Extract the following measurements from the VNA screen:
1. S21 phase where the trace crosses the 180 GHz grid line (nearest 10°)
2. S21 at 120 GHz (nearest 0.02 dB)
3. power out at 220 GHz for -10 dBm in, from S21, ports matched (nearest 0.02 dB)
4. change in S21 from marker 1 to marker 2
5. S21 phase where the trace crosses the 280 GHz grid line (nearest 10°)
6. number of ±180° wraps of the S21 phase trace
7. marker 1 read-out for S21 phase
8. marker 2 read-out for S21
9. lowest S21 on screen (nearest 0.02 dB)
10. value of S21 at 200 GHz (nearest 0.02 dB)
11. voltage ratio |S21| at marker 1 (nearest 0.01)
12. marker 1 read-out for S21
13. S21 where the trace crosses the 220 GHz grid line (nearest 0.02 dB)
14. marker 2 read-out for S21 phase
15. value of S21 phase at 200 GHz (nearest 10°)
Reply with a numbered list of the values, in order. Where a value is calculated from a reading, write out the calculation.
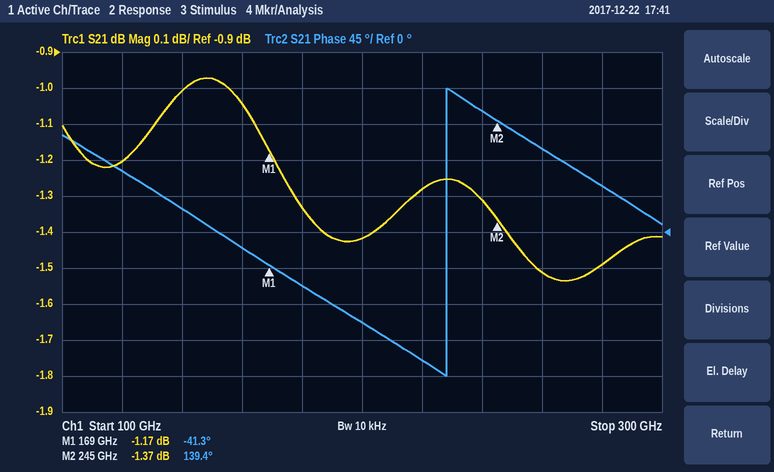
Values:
1. -70°
2. -1.20 dB
3. -10 dBm + (-1.28 dB) = -11.28 dBm
4. -1.37 − (-1.17) = -0.20 dB
5. 60°
6. 1
7. -41.3°
8. -1.37 dB
9. -1.54 dB
10. -1.42 dB
11. 10^(-1.17/20) ≈ 0.87
12. -1.17 dB
13. -1.28 dB
14. 139.4°
15. -110°
